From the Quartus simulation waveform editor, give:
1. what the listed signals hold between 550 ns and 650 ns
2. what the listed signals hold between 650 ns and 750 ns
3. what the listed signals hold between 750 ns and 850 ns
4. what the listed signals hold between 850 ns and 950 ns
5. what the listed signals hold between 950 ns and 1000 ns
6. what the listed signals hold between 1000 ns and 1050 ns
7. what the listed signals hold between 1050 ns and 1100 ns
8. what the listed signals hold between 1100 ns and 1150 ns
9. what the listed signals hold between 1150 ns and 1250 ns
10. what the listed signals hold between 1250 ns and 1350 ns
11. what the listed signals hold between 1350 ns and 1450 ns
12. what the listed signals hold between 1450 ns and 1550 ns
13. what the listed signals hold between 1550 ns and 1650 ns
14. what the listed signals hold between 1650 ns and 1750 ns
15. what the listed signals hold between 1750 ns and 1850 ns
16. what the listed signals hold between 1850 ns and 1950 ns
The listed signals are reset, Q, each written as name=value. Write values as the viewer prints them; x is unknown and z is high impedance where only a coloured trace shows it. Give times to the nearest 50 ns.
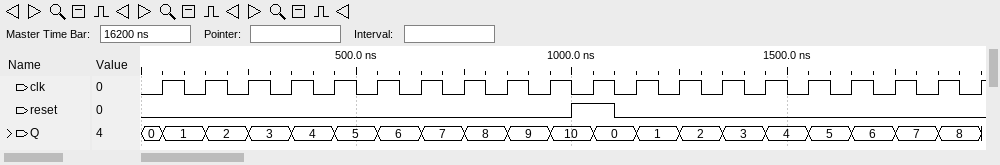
reset=0, Q=6
reset=0, Q=7
reset=0, Q=8
reset=0, Q=9
reset=0, Q=10
reset=1, Q=10
reset=1, Q=0
reset=0, Q=0
reset=0, Q=1
reset=0, Q=2
reset=0, Q=3
reset=0, Q=4
reset=0, Q=5
reset=0, Q=6
reset=0, Q=7
reset=0, Q=8
